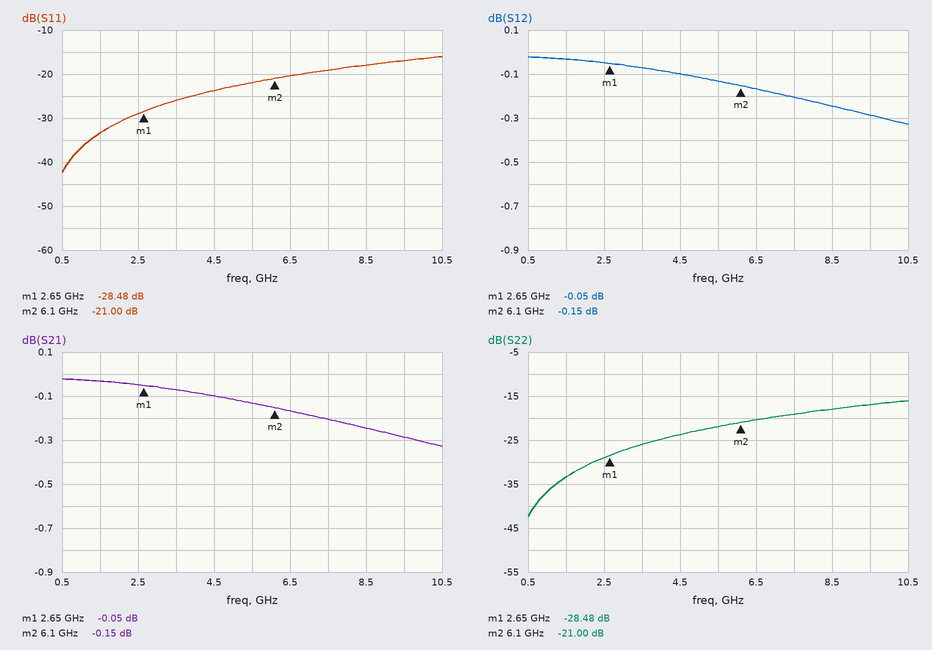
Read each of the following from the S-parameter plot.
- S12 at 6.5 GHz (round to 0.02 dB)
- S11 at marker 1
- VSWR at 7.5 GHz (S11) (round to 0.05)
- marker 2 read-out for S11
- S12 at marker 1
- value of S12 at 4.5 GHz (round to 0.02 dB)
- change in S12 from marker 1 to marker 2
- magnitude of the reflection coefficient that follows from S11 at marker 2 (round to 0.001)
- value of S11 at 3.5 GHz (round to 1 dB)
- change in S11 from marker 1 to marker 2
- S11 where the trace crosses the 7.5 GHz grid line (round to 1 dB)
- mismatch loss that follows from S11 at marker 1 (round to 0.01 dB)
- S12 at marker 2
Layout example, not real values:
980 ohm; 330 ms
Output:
-0.16 dB; -28.48 dB; 1.25; -21.00 dB; -0.05 dB; -0.10 dB; -0.10 dB; 0.089; -26 dB; 7.48 dB; -19 dB; 0.01 dB; -0.15 dB
